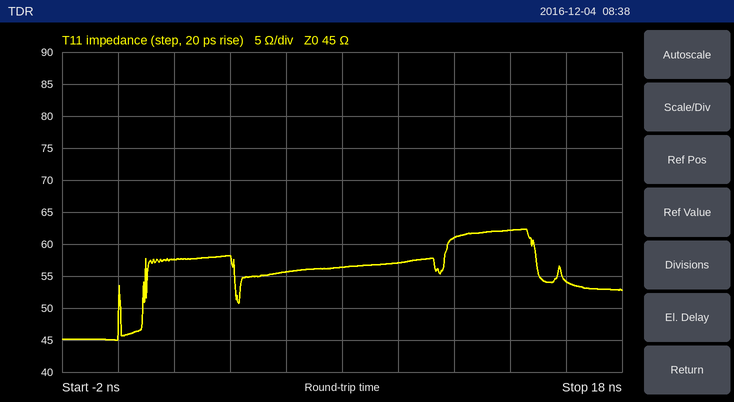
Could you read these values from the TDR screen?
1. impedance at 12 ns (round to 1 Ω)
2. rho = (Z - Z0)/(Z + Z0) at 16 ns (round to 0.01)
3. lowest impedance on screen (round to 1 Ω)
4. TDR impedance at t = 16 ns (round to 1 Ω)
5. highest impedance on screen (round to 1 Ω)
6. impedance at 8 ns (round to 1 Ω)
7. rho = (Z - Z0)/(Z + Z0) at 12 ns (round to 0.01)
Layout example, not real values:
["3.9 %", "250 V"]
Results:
["61 Ω", "+0.09", "45 Ω", "54 Ω", "62 Ω", "56 Ω", "+0.15"]
